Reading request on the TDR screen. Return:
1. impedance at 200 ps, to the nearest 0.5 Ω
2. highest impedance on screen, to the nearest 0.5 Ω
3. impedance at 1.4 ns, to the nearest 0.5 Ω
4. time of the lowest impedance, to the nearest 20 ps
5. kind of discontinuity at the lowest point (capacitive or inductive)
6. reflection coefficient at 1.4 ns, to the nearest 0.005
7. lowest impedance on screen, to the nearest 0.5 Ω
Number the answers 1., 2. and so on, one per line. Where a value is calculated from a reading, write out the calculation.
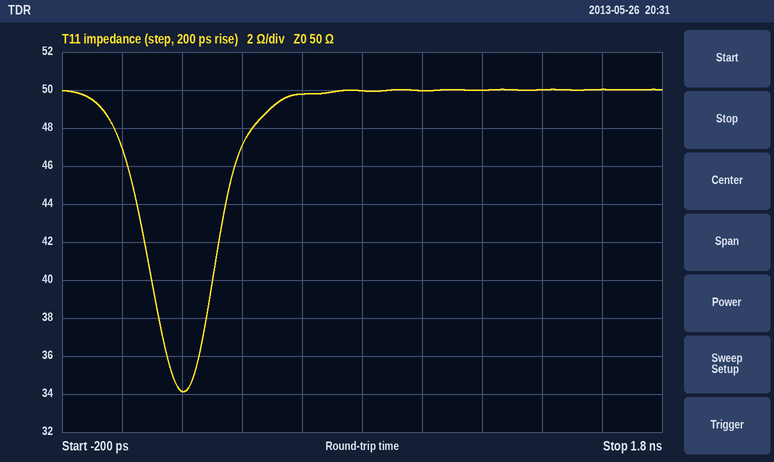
1. 34.0 Ω
2. 50.0 Ω
3. 50.0 Ω
4. 200 ps
5. capacitive
6. (50 − 50)/(50 + 50) ≈ 0.000
7. 34.0 Ω
